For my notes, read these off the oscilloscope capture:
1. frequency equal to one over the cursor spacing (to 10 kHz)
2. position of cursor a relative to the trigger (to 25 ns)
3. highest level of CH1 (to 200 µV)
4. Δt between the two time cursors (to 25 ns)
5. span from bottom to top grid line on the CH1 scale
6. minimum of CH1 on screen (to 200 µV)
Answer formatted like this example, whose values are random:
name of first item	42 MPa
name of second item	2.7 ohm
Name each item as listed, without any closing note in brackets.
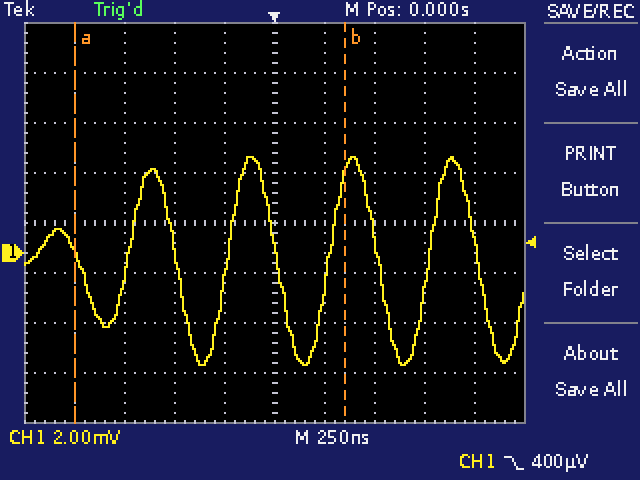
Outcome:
frequency equal to one over the cursor spacing	740 kHz
position of cursor a relative to the trigger	-1.000 µs
highest level of CH1	3.8 mV
Δt between the two time cursors	1.350 µs
span from bottom to top grid line on the CH1 scale	16 mV
minimum of CH1 on screen	-4.4 mV
